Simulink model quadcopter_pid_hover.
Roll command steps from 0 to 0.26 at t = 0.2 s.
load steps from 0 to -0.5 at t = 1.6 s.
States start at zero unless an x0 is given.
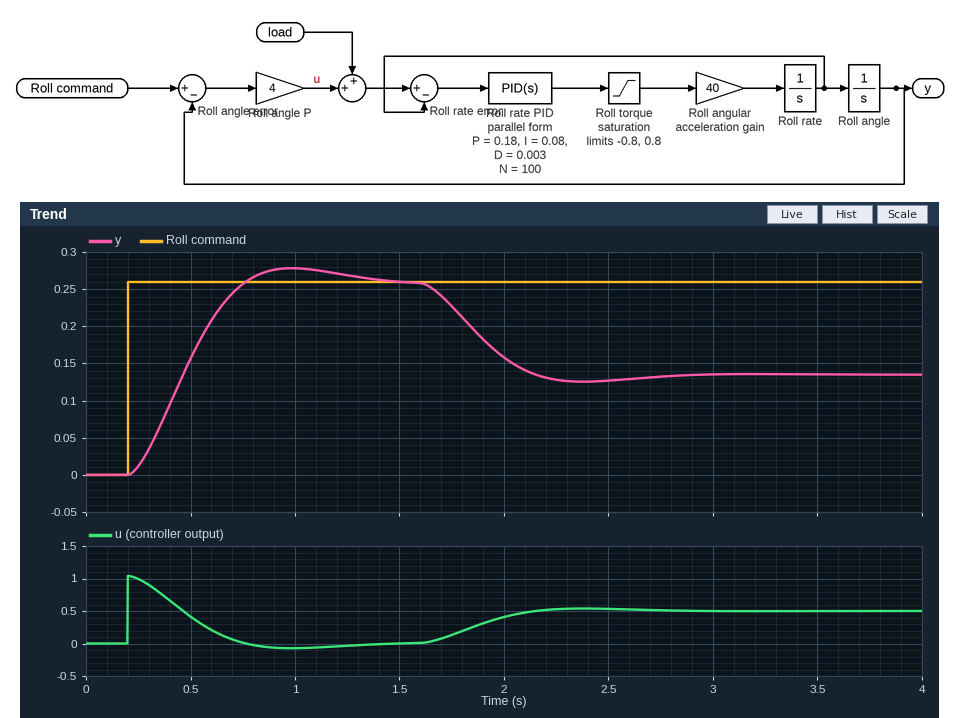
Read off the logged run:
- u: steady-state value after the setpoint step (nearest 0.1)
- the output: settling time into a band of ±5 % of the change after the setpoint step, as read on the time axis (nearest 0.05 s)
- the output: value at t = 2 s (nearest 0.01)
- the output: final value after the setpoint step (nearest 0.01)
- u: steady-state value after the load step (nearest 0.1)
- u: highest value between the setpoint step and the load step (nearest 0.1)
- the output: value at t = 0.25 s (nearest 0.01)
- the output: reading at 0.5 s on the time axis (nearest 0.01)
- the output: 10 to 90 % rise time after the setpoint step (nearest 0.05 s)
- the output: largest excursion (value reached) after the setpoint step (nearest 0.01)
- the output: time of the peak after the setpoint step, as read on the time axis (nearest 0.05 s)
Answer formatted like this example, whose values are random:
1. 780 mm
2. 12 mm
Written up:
1. 0.0
2. 1.15 s
3. 0.16
4. 0.26
5. 0.5
6. 1.0
7. 0.01
8. 0.16
9. 0.40 s
10. 0.28
11. 1.00 s
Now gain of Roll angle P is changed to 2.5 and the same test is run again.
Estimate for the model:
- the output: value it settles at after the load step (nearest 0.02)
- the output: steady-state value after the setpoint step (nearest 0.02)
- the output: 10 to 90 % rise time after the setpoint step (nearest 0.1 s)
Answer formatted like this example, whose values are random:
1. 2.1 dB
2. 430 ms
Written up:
1. 0.06
2. 0.26
3. 0.6 s
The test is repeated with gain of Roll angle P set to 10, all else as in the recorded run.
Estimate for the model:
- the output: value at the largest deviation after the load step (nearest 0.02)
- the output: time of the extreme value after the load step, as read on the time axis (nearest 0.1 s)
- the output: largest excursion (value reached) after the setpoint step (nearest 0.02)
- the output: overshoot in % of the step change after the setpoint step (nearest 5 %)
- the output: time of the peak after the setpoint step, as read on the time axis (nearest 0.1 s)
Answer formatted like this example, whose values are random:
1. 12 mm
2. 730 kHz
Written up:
1. 0.20
2. 2.0 s
3. 0.32
4. 20 %
5. 0.6 s
